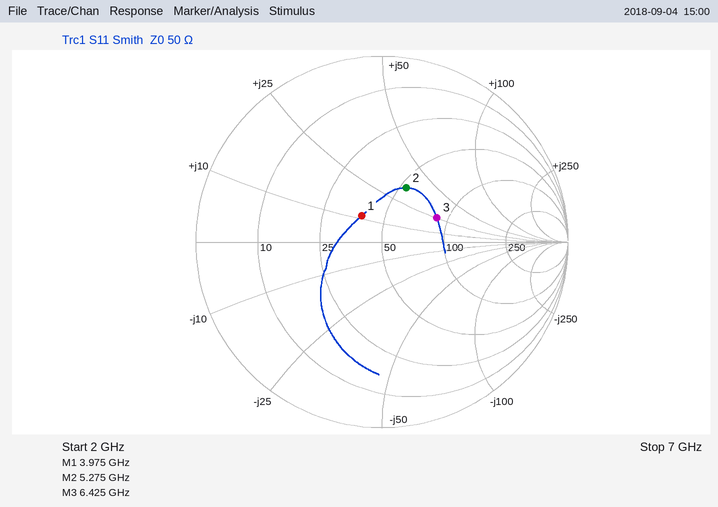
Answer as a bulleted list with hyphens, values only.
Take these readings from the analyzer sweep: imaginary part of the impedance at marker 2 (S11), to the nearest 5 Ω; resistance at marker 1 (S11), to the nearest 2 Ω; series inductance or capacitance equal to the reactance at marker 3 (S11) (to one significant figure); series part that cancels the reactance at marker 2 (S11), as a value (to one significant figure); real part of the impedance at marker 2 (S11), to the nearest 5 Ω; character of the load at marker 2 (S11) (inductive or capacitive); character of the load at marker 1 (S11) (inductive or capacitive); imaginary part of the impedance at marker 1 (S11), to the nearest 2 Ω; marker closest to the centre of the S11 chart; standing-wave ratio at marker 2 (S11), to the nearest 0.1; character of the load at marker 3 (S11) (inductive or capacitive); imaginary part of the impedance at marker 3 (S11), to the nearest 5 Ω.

- +35 Ω
- 38 Ω
- 600 pH
- 900 fF
- 55 Ω
- inductive
- inductive
- +12 Ω
- marker 1
- 1.9
- inductive
- +25 Ω
